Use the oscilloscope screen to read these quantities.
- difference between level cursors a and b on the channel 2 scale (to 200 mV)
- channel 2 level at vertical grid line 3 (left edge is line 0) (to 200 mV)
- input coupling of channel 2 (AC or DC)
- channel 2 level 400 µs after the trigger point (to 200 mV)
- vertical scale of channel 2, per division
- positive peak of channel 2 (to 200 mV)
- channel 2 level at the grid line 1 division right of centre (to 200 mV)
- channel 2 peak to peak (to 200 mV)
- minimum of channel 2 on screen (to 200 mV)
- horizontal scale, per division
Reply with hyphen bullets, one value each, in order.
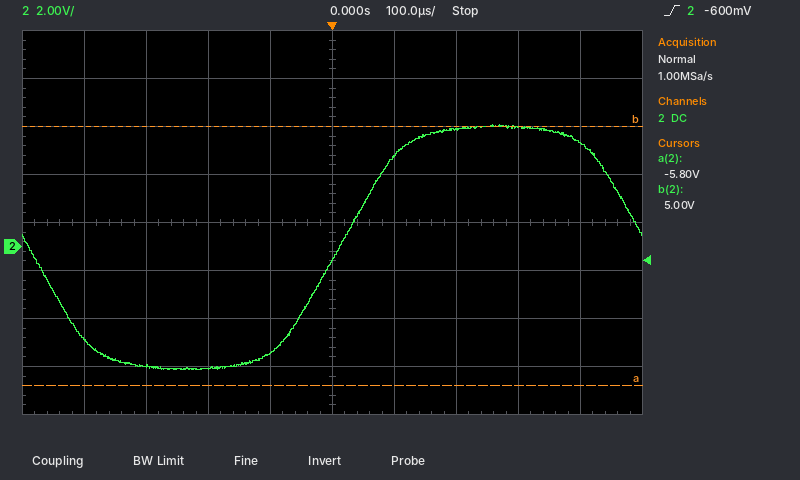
- 10.8 V
- -5.0 V
- DC
- 4.4 V
- 2 V
- 5.0 V
- 3.8 V
- 10.2 V
- -5.2 V
- 100 µs
